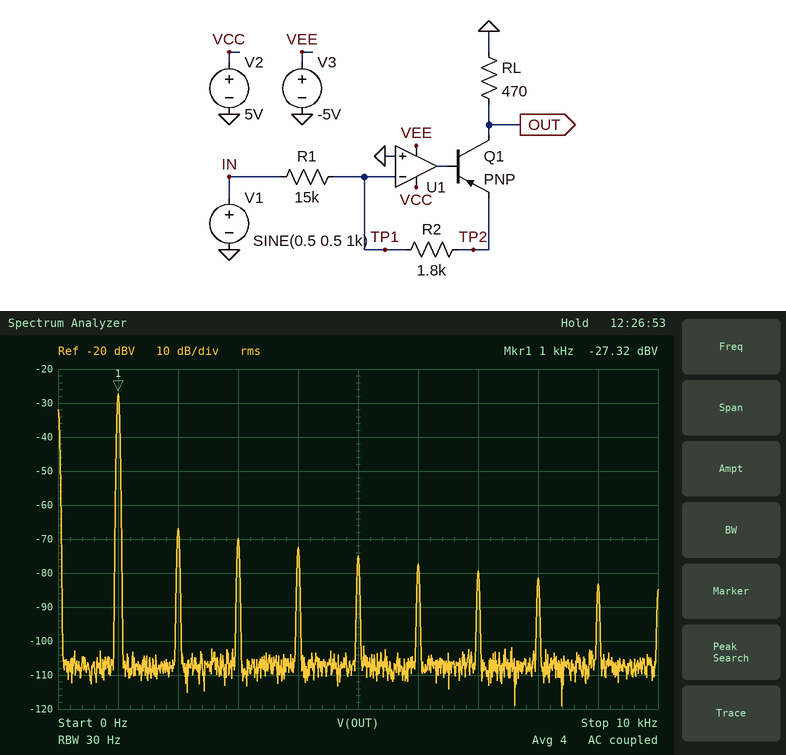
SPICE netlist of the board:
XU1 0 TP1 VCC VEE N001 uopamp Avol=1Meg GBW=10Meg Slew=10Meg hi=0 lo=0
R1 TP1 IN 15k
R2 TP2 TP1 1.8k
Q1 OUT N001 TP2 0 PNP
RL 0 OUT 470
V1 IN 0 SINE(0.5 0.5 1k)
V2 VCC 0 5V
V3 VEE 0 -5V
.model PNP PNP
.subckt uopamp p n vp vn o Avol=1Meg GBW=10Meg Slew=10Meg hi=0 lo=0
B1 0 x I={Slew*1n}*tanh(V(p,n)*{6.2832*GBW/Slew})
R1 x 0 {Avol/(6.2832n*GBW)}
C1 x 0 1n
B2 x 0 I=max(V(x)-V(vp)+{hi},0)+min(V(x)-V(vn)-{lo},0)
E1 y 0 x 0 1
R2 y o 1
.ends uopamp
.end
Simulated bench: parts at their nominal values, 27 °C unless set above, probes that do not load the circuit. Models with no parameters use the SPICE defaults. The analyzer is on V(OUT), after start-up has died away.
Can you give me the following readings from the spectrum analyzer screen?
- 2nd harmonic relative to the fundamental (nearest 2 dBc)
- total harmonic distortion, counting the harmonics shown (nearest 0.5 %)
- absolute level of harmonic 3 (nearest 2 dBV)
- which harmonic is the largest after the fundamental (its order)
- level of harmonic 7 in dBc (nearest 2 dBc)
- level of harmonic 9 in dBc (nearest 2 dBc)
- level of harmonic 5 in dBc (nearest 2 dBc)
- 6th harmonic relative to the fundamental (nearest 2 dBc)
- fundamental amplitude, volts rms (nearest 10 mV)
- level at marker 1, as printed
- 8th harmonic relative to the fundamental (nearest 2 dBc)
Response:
-40 dBc
1.5 %
-70 dBV
2
-52 dBc
-56 dBc
-48 dBc
-50 dBc
40 mV
-27.32 dBV
-54 dBc
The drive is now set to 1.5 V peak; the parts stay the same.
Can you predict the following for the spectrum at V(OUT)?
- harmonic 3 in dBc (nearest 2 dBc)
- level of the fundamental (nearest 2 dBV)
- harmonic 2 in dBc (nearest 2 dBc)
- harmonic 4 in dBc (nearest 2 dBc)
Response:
-22 dBc
-20 dBV
-12 dBc
-38 dBc
